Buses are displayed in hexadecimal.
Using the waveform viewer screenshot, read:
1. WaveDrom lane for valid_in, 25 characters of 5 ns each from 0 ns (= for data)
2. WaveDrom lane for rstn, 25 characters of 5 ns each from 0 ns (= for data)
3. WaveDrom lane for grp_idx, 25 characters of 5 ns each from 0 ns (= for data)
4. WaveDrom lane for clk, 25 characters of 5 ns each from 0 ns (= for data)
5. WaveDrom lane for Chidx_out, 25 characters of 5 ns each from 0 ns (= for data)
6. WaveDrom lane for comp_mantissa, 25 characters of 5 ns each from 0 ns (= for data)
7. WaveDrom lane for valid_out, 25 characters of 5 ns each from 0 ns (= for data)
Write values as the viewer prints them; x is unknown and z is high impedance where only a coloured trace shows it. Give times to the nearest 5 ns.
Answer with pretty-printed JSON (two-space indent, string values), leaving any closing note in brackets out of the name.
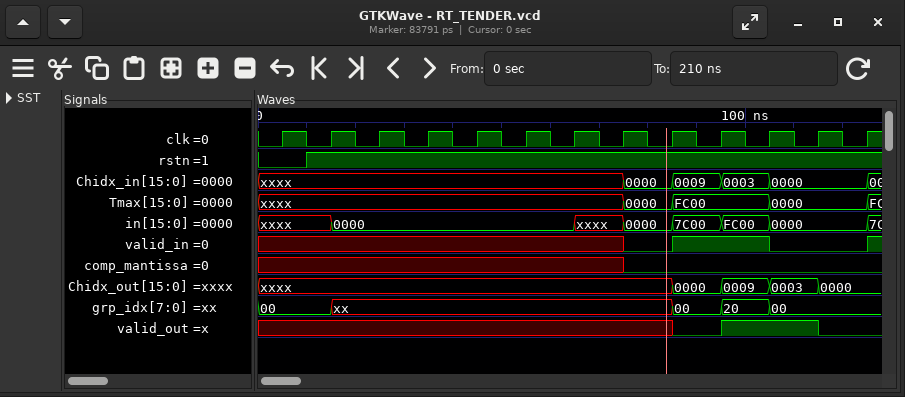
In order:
{
  "WaveDrom lane for valid_in, 25 characters of 5 ns each from 0 ns": "{name: 'valid_in', wave: 'x..............0.1...0...'}",
  "WaveDrom lane for rstn, 25 characters of 5 ns each from 0 ns": "{name: 'rstn', wave: '0.1......................'}",
  "WaveDrom lane for grp_idx, 25 characters of 5 ns each from 0 ns": "{name: 'grp_idx', wave: '=..x.............=.=.=...', data: '00 00 20 00'}",
  "WaveDrom lane for clk, 25 characters of 5 ns each from 0 ns": "{name: 'clk', wave: '0101010101010101010101010'}",
  "WaveDrom lane for Chidx_out, 25 characters of 5 ns each from 0 ns": "{name: 'Chidx_out', wave: 'x................=.=.=.=.', data: '0000 0009 0003 0000'}",
  "WaveDrom lane for comp_mantissa, 25 characters of 5 ns each from 0 ns": "{name: 'comp_mantissa', wave: 'x..............0.........'}",
  "WaveDrom lane for valid_out, 25 characters of 5 ns each from 0 ns": "{name: 'valid_out', wave: 'x................0.1...0.'}"
}
